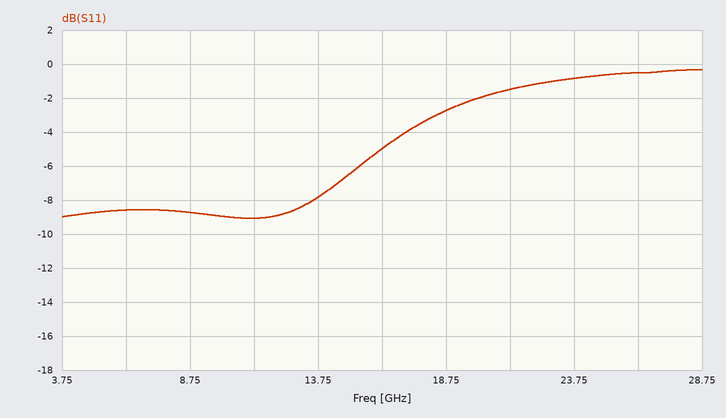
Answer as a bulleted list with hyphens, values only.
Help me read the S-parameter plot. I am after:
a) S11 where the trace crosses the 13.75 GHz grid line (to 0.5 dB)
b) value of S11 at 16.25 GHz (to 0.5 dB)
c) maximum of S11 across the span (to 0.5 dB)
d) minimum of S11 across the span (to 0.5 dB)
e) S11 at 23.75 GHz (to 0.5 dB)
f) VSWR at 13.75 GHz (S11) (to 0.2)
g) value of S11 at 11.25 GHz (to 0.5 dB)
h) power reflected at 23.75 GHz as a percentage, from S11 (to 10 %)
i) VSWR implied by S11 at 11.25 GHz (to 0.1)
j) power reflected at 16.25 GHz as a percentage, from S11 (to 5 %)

- -8.0 dB
- -5.0 dB
- -0.5 dB
- -9.0 dB
- -1.0 dB
- 2.4
- -9.0 dB
- 80 %
- 2.1
- 30 %
